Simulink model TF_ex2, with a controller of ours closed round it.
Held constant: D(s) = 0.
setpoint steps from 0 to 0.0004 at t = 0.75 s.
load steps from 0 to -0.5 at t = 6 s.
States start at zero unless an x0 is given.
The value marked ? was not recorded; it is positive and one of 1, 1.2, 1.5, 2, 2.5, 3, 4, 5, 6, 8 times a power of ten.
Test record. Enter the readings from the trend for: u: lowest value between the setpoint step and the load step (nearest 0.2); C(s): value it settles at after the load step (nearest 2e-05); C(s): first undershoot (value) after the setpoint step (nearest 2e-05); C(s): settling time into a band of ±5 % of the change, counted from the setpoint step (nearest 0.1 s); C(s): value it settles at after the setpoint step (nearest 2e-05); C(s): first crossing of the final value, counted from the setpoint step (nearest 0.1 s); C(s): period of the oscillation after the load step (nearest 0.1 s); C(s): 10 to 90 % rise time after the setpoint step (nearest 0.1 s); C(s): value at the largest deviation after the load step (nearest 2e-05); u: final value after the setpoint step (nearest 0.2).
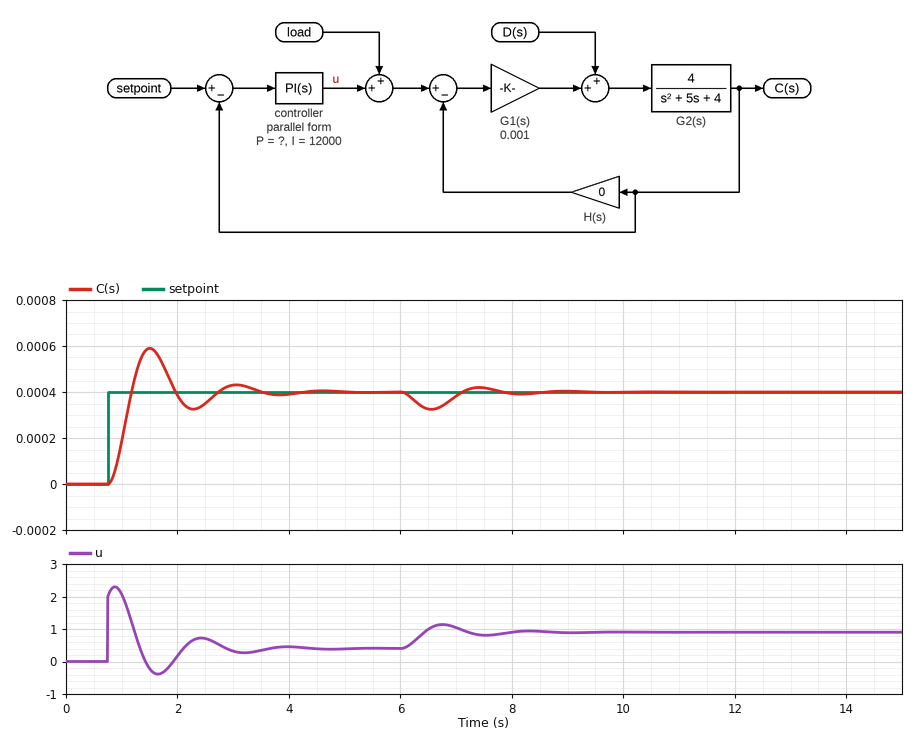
-0.4
0.00040
0.00032
2.5 s
0.00040
0.4 s
1.6 s
0.3 s
0.00032
0.4
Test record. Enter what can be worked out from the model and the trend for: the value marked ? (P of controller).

5000
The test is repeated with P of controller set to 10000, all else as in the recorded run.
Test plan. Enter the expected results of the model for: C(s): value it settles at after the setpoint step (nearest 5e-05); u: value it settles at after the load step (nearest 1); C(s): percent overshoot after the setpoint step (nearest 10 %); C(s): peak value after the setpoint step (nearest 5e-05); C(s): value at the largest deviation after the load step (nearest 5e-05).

0.00040
1
40 %
0.00055
0.00035
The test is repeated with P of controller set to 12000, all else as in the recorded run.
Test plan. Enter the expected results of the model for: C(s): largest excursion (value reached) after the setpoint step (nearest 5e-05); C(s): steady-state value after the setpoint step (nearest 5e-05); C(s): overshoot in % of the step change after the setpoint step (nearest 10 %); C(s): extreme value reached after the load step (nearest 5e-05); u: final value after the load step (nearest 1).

0.00055
0.00040
40 %
0.00035
1
